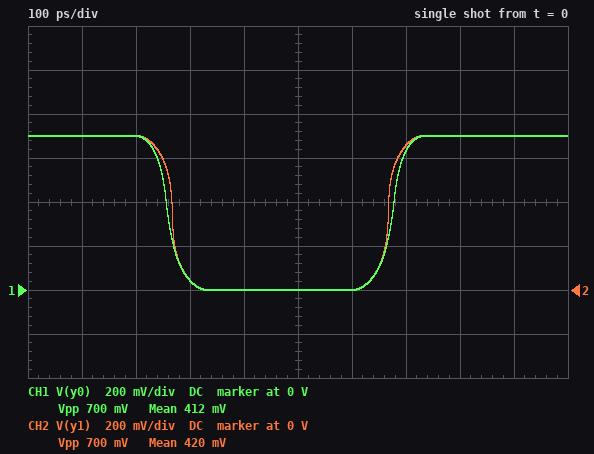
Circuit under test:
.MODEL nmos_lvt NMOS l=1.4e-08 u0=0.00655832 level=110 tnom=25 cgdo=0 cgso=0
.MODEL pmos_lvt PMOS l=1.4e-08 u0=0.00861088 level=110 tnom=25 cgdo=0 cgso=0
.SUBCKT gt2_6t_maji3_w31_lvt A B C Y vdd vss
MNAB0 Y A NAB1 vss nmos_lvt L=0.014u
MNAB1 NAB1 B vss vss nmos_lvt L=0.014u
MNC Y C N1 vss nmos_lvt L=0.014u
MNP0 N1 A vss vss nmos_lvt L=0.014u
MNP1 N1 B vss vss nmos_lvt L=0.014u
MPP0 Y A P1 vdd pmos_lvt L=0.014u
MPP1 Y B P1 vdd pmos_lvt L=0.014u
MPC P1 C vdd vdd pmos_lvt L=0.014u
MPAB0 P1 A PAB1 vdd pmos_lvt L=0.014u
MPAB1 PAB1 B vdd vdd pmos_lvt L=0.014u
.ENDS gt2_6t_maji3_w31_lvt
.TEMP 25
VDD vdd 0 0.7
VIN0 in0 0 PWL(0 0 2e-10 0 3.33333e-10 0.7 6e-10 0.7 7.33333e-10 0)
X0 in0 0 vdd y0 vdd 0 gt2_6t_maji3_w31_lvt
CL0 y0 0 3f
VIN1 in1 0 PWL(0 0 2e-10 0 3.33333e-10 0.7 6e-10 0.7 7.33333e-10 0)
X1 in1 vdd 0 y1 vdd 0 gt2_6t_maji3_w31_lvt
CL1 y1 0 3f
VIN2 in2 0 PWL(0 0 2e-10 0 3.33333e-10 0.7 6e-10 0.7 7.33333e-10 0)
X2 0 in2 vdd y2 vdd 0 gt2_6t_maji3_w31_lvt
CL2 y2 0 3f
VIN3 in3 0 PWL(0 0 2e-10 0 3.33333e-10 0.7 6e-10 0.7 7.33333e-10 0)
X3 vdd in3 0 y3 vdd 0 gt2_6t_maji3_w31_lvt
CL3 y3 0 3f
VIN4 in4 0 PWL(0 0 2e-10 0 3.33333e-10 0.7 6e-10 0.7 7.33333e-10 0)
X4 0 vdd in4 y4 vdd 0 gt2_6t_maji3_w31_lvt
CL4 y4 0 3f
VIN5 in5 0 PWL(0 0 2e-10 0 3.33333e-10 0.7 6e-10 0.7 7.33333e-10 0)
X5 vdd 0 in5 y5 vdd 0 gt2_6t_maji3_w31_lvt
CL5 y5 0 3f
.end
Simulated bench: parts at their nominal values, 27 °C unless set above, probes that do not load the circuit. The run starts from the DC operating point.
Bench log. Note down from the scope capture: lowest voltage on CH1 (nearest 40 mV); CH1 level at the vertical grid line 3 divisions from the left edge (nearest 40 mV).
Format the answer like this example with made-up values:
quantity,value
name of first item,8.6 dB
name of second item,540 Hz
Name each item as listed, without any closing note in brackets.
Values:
quantity,value
lowest voltage on CH1,0 V
CH1 level at the vertical grid line 3 divisions from the left edge,40 mV
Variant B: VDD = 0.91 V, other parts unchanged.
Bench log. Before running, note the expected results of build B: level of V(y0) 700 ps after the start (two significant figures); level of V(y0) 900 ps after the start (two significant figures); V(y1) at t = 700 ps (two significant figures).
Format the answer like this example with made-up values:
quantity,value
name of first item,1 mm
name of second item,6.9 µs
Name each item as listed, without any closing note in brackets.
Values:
quantity,value
level of V(y0) 700 ps after the start,860 mV
level of V(y0) 900 ps after the start,910 mV
V(y1) at t = 700 ps,880 mV
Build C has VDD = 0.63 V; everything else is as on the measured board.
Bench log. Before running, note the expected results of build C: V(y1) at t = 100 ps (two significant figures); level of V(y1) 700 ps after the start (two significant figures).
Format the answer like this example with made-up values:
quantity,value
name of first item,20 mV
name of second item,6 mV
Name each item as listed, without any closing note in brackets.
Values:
quantity,value
V(y1) at t = 100 ps,630 mV
level of V(y1) 700 ps after the start,580 mV
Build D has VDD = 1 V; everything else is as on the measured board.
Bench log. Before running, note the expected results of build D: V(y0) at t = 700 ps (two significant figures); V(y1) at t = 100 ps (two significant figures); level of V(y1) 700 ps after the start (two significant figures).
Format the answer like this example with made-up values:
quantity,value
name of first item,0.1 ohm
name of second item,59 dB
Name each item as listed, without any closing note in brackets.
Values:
quantity,value
V(y0) at t = 700 ps,960 mV
V(y1) at t = 100 ps,1.0 V
level of V(y1) 700 ps after the start,970 mV
